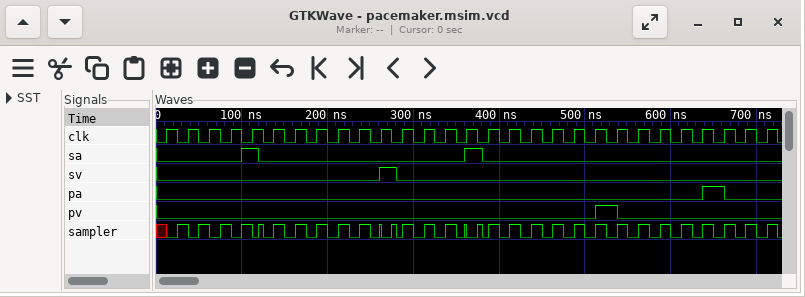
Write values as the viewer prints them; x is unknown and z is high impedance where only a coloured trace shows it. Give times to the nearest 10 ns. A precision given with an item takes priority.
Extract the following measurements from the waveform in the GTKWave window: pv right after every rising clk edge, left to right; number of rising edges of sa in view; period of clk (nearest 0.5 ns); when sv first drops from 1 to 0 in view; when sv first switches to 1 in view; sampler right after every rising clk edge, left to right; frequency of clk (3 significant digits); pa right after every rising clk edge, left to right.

0 0 0 0 0 0 0 0 0 0 0 0 0 0 0 0 0 0 0 0 1 0 0 0 0 0 0 0 0
2
25 ns
280 ns
260 ns
0 0 0 0 0 1 1 1 1 1 0 1 1 1 0 1 1 1 1 1 1 1 1 1 1 1 1 1 1
40.0 MHz
0 0 0 0 0 0 0 0 0 0 0 0 0 0 0 0 0 0 0 0 0 0 0 0 0 1 0 0 0
